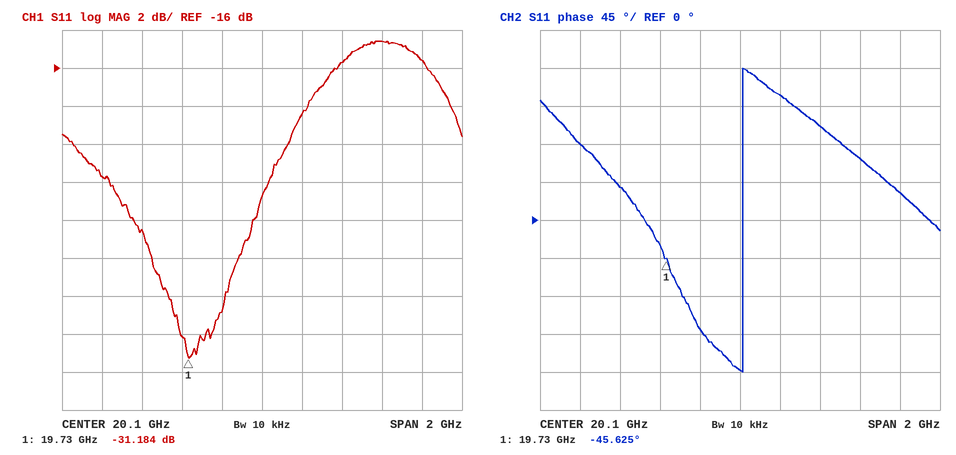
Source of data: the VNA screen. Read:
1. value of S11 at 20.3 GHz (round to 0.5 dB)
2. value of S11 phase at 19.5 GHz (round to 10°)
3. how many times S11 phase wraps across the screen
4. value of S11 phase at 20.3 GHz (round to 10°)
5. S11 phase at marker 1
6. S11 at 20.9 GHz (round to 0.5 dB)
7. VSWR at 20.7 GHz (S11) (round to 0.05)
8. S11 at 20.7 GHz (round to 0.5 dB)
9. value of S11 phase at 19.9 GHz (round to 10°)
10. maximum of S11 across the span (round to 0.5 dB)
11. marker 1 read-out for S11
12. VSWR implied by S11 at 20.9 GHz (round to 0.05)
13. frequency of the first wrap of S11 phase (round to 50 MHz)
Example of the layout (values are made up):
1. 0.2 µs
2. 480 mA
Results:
1. -18.5 dB
2. 40°
3. 1
4. 150°
5. -45.625°
6. -15.5 dB
7. 1.45
8. -14.5 dB
9. -130°
10. -14.5 dB
11. -31.184 dB
12. 1.40
13. 20.10 GHz
